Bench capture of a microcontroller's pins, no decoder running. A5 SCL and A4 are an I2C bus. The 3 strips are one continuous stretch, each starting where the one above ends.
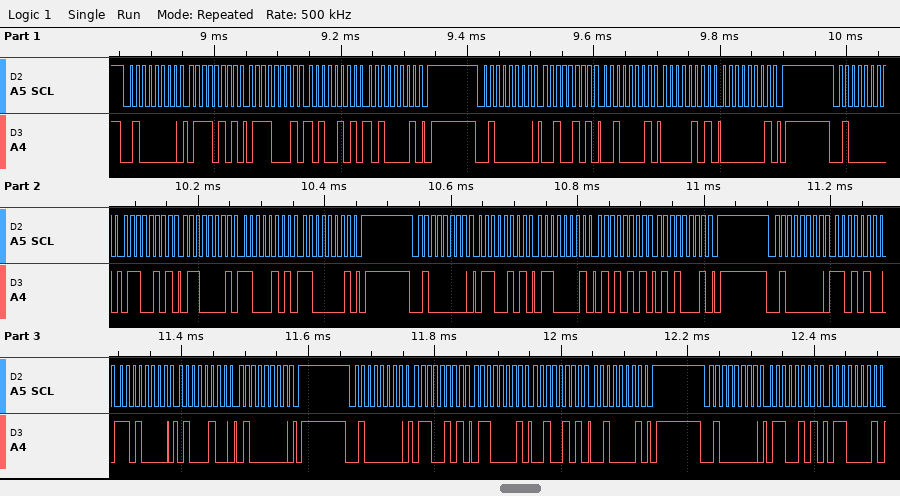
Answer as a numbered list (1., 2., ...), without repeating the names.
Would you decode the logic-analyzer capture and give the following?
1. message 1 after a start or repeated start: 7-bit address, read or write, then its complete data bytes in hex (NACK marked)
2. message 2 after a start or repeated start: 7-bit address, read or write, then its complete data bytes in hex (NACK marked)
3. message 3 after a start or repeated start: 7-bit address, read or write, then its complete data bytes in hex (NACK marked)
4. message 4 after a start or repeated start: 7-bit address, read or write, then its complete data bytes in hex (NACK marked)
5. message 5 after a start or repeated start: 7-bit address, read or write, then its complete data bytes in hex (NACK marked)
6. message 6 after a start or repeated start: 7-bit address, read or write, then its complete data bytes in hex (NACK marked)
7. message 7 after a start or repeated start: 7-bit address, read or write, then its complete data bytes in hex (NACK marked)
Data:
1. 0x20 write: 75 71 A5 A1
2. 0x20 write: 25 21 05 01
3. 0x20 write: 65 61 C5 C1
4. 0x20 write: 65 61 55 51
5. 0x20 write: D4 D0 44 40
6. 0x20 write: 65 61 25 21
7. 0x20 write: 65 61
